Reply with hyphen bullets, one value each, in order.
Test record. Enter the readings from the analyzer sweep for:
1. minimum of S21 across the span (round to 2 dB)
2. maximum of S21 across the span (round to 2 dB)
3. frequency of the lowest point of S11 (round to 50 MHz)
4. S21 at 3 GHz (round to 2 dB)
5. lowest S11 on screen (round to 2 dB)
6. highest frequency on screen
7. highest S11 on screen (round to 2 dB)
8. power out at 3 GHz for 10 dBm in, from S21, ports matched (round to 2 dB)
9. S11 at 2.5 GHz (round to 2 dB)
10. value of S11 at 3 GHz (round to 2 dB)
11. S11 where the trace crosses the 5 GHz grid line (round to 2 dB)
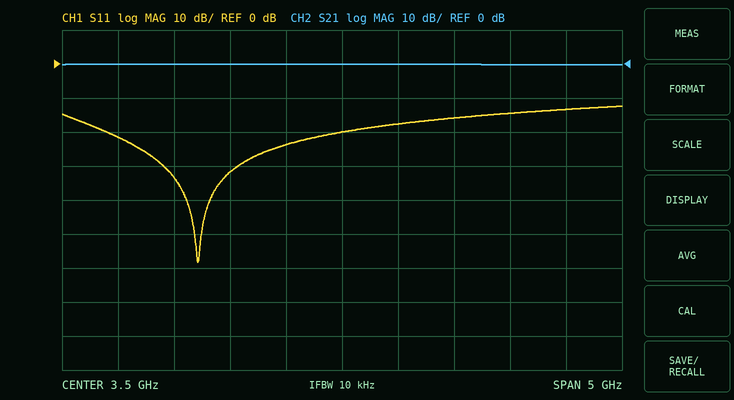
- 0 dB
- 0 dB
- 2.20 GHz
- 0 dB
- -58 dB
- 6 GHz
- -12 dB
- 10 dBm
- -32 dB
- -24 dB
- -14 dB
